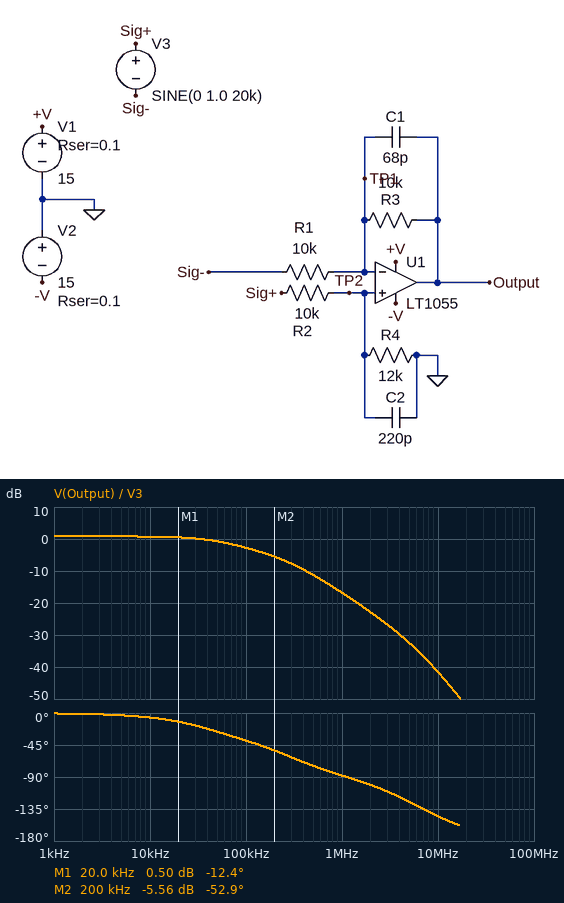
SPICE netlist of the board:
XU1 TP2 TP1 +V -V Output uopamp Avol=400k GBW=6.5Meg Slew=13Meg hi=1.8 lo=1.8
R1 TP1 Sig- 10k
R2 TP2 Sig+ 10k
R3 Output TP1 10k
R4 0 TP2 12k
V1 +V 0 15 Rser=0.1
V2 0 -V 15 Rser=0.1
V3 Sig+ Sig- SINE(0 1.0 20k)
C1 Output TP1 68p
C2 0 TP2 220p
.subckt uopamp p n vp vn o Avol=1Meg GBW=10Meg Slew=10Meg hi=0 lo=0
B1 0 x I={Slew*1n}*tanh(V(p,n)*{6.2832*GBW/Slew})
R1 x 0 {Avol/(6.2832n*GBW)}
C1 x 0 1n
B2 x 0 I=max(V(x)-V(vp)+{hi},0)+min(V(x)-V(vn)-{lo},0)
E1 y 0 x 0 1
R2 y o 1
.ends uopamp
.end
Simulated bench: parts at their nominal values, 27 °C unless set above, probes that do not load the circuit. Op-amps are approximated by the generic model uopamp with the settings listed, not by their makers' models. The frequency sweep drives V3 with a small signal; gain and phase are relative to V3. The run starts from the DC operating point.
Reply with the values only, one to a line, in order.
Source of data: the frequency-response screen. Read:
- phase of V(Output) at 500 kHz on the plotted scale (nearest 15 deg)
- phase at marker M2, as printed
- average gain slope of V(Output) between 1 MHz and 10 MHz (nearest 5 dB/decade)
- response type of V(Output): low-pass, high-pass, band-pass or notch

-75 deg
-52.9 deg
-25 dB/decade
low-pass
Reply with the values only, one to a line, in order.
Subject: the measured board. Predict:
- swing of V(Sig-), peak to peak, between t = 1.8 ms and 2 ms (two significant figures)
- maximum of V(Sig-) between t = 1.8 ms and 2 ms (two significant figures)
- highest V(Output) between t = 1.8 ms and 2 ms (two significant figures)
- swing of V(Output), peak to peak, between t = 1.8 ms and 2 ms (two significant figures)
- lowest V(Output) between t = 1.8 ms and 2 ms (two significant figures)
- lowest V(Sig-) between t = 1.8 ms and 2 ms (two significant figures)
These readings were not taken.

370 mV
190 mV
1.1 V
2.1 V
-1.1 V
-190 mV
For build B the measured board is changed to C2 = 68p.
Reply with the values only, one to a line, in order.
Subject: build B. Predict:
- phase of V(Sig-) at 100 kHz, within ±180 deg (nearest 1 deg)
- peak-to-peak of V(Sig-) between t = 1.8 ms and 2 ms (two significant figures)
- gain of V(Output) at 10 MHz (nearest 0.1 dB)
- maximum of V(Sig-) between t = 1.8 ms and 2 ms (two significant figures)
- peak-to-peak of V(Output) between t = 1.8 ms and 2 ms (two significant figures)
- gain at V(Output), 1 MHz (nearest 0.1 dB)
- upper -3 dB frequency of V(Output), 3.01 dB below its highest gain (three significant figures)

-98 deg
230 mV
-38.0 dB
110 mV
2.2 V
-13.2 dB
203 kHz
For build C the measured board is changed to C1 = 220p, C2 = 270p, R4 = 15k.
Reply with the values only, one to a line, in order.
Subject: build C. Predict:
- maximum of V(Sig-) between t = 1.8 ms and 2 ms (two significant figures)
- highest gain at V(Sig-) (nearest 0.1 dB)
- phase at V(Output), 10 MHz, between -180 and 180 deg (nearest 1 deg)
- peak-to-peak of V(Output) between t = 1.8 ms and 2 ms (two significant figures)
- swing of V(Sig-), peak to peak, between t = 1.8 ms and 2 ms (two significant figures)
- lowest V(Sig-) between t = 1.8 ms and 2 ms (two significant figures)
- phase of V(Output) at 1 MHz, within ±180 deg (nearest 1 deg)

320 mV
-5.9 dB
-146 deg
2.3 V
640 mV
-320 mV
-95 deg
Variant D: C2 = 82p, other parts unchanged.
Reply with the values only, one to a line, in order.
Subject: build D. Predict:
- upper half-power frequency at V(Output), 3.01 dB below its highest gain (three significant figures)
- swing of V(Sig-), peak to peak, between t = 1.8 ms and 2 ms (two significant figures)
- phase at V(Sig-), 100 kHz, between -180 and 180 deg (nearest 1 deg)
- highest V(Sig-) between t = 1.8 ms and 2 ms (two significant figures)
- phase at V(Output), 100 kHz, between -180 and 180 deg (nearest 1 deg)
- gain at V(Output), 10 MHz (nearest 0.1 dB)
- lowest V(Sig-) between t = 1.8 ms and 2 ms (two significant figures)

182 kHz
240 mV
-105 deg
120 mV
-29 deg
-38.7 dB
-120 mV
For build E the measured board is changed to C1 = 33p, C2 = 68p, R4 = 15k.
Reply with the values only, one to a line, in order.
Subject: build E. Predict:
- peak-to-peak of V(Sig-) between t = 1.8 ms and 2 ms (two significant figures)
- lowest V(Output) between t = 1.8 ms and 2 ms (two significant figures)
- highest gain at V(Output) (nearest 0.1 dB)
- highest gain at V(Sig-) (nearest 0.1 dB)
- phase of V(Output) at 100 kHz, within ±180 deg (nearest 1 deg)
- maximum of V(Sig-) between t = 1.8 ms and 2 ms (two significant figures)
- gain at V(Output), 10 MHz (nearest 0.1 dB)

510 mV
-1.2 V
1.9 dB
-5.6 dB
-25 deg
260 mV
-34.3 dB
